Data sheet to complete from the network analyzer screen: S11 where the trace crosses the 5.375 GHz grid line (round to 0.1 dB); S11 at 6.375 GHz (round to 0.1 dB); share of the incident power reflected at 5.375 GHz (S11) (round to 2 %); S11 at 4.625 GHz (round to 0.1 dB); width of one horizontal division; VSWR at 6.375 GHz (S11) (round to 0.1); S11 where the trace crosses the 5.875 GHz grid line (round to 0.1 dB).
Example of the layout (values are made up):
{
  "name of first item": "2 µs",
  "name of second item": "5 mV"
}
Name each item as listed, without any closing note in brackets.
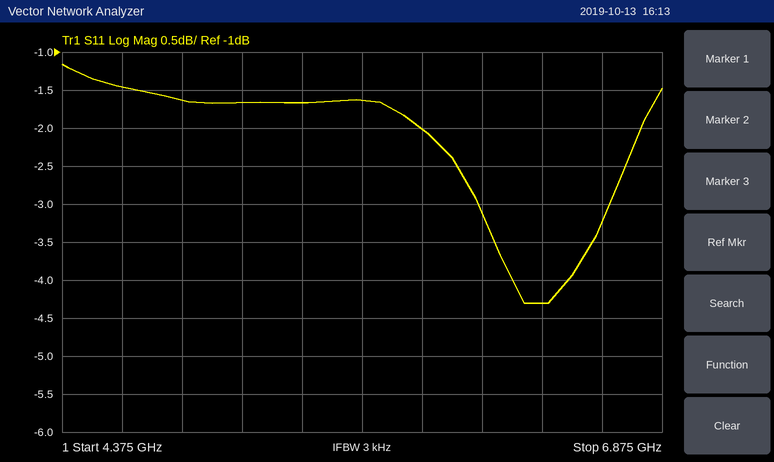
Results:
{
  "S11 where the trace crosses the 5.375 GHz grid line": "-1.7 dB",
  "S11 at 6.375 GHz": "-4.3 dB",
  "share of the incident power reflected at 5.375 GHz (S11)": "68 %",
  "S11 at 4.625 GHz": "-1.5 dB",
  "width of one horizontal division": "250 MHz",
  "VSWR at 6.375 GHz (S11)": "4.1",
  "S11 where the trace crosses the 5.875 GHz grid line": "-2.0 dB"
}
